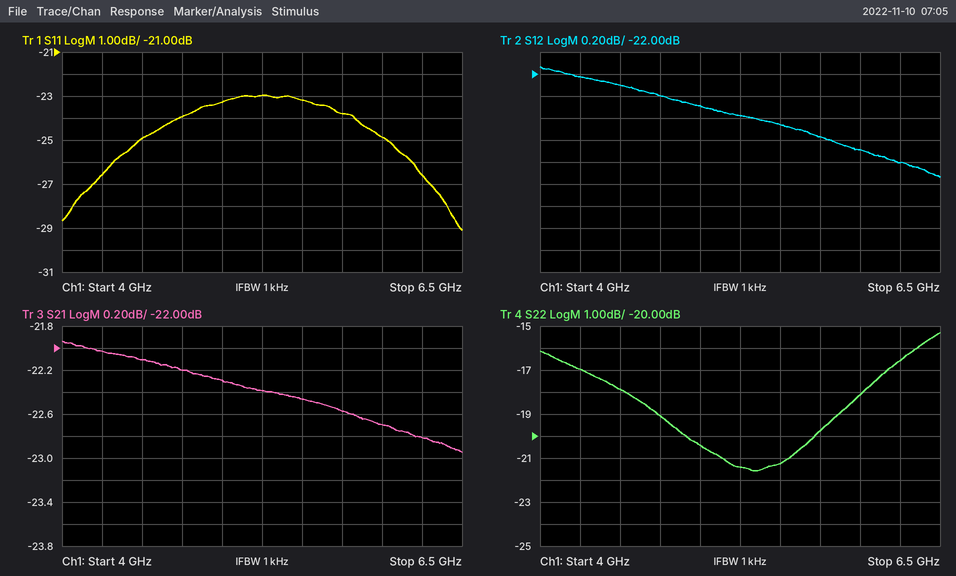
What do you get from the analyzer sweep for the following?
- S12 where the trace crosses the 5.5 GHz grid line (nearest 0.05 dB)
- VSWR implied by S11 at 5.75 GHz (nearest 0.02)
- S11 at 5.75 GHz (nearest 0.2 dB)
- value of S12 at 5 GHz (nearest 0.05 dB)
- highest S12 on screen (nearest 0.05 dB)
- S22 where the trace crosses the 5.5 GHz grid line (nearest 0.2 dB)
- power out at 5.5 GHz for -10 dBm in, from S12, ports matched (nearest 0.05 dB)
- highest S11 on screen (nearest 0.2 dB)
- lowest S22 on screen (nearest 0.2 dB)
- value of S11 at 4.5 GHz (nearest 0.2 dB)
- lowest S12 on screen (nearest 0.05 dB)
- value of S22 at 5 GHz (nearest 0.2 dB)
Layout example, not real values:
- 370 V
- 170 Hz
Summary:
- -22.45 dB
- 1.14
- -23.8 dB
- -22.30 dB
- -21.95 dB
- -21.2 dB
- -32.45 dBm
- -23.0 dB
- -21.6 dB
- -25.0 dB
- -22.95 dB
- -20.4 dB
